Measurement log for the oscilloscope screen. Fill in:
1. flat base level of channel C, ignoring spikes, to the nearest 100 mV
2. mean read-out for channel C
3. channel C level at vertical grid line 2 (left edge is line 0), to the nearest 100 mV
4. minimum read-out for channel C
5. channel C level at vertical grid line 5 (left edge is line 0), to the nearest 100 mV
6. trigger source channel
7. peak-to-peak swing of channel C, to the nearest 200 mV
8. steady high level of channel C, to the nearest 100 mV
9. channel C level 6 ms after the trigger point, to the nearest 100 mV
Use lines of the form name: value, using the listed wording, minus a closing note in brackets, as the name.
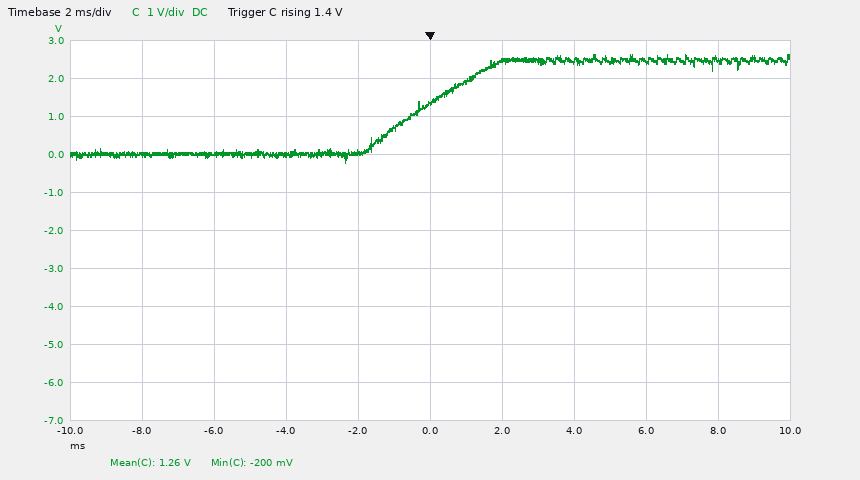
flat base level of channel C, ignoring spikes, to the nearest 100 mV: 0.0 V
mean read-out for channel C: 1.26 V
channel C level at vertical grid line 2 (left edge is line 0), to the nearest 100 mV: 0.0 V
minimum read-out for channel C: -200 mV
channel C level at vertical grid line 5 (left edge is line 0), to the nearest 100 mV: 1.4 V
trigger source channel: channel C
peak-to-peak swing of channel C, to the nearest 200 mV: 2.8 V
steady high level of channel C, to the nearest 100 mV: 2.5 V
channel C level 6 ms after the trigger point, to the nearest 100 mV: 2.5 V
